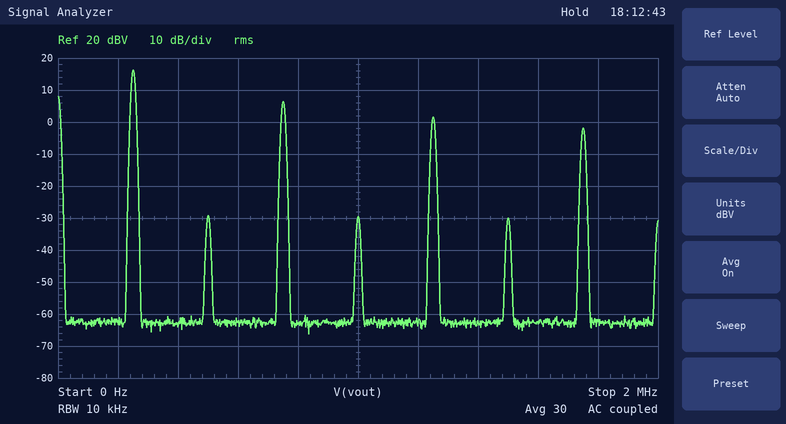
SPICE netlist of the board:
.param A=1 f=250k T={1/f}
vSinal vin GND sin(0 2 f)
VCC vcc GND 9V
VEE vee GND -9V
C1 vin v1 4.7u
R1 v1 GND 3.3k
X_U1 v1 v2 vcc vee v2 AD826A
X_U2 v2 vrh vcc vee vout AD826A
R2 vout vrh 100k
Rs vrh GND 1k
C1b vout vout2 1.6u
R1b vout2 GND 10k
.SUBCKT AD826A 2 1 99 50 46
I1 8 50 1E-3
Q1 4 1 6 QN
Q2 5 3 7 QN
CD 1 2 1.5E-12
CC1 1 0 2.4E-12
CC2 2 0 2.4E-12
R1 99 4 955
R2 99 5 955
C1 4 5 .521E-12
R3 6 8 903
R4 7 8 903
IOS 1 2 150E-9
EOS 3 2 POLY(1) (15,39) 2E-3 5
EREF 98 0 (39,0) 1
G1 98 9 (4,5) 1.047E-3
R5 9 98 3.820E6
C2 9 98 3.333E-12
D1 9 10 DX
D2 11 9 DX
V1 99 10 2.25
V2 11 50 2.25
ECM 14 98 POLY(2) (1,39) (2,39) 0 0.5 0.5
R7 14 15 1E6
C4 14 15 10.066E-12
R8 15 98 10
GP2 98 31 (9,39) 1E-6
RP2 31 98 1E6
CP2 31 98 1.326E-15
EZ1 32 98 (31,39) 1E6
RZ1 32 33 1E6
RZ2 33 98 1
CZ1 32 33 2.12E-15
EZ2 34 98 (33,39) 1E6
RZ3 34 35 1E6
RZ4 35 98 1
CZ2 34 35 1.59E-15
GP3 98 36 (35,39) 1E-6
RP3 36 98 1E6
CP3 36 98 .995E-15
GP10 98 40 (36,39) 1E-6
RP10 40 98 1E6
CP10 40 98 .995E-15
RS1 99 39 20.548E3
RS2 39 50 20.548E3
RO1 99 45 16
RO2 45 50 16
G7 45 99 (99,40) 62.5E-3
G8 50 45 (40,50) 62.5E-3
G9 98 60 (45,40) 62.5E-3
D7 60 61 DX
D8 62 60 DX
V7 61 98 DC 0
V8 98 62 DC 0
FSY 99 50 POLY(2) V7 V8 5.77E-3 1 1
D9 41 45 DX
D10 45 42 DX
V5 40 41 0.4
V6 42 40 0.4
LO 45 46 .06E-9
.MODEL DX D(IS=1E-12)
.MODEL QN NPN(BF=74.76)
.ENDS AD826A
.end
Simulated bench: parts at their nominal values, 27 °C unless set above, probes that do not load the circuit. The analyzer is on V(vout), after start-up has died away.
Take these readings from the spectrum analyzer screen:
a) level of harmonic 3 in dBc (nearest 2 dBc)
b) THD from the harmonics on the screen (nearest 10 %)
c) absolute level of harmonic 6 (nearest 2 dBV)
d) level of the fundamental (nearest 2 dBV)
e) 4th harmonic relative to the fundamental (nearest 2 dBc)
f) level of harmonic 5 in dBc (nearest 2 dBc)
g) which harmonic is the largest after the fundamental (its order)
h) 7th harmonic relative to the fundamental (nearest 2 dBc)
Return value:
-10 dBc
40 %
-30 dBV
16 dBV
-46 dBc
-14 dBc
3
-18 dBc
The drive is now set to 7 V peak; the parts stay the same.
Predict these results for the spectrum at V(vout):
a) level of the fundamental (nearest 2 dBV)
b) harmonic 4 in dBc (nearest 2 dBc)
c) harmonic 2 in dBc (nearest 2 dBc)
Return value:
16 dBV
-56 dBc
-56 dBc
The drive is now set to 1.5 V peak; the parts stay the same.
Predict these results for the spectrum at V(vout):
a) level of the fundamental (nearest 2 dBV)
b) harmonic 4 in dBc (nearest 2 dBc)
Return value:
16 dBV
-44 dBc
